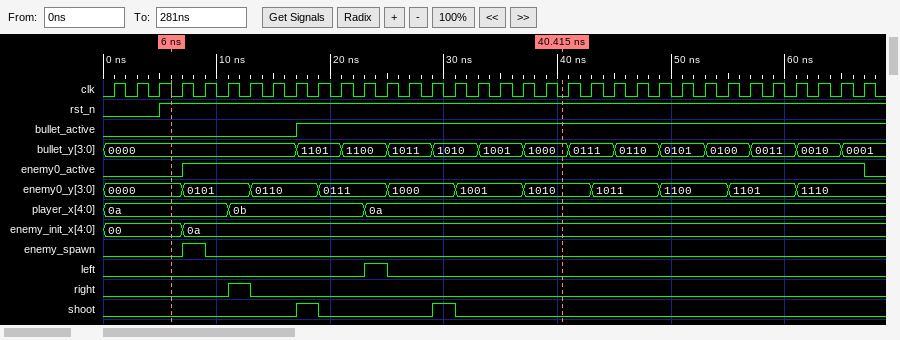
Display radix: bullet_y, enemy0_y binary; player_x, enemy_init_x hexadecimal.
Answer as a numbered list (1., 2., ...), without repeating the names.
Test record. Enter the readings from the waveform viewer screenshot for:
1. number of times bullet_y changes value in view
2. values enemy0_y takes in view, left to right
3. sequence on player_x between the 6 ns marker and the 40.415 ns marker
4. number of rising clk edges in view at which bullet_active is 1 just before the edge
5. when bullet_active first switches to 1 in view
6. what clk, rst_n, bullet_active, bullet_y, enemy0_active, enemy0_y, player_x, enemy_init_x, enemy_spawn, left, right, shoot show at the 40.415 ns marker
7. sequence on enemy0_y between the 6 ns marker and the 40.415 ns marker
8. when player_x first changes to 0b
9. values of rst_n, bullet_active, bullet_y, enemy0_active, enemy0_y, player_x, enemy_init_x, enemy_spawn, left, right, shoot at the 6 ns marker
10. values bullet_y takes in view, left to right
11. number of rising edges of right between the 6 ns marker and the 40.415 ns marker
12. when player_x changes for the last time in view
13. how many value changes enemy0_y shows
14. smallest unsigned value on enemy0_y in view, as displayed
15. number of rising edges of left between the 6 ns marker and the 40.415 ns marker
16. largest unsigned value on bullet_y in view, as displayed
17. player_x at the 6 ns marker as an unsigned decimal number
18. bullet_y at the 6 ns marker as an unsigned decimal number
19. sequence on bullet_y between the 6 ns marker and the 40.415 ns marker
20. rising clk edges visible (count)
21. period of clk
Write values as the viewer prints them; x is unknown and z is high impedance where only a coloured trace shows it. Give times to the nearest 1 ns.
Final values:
1. 13
2. 0000, 0101, 0110, 0111, 1000, 1001, 1010, 1011, 1100, 1101, 1110
3. 0a, 0b, 0a
4. 25
5. 17 ns
6. clk=0, rst_n=1, bullet_active=1, bullet_y=1000, enemy0_active=1, enemy0_y=1010, player_x=0a, enemy_init_x=0a, enemy_spawn=0, left=0, right=0, shoot=0
7. 0000, 0101, 0110, 0111, 1000, 1001, 1010
8. 11 ns
9. rst_n=1, bullet_active=0, bullet_y=0000, enemy0_active=0, enemy0_y=0000, player_x=0a, enemy_init_x=00, enemy_spawn=0, left=0, right=0, shoot=0
10. 0000, 1101, 1100, 1011, 1010, 1001, 1000, 0111, 0110, 0101, 0100, 0011, 0010, 0001
11. 1
12. 23 ns
13. 10
14. 0000
15. 1
16. 1101
17. 10
18. 0
19. 0000, 1101, 1100, 1011, 1010, 1001, 1000
20. 34
21. 2 ns
